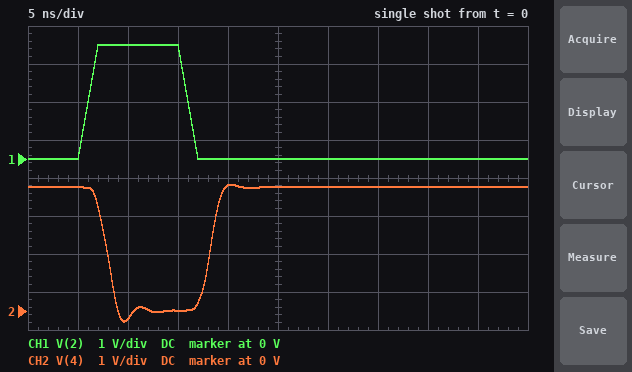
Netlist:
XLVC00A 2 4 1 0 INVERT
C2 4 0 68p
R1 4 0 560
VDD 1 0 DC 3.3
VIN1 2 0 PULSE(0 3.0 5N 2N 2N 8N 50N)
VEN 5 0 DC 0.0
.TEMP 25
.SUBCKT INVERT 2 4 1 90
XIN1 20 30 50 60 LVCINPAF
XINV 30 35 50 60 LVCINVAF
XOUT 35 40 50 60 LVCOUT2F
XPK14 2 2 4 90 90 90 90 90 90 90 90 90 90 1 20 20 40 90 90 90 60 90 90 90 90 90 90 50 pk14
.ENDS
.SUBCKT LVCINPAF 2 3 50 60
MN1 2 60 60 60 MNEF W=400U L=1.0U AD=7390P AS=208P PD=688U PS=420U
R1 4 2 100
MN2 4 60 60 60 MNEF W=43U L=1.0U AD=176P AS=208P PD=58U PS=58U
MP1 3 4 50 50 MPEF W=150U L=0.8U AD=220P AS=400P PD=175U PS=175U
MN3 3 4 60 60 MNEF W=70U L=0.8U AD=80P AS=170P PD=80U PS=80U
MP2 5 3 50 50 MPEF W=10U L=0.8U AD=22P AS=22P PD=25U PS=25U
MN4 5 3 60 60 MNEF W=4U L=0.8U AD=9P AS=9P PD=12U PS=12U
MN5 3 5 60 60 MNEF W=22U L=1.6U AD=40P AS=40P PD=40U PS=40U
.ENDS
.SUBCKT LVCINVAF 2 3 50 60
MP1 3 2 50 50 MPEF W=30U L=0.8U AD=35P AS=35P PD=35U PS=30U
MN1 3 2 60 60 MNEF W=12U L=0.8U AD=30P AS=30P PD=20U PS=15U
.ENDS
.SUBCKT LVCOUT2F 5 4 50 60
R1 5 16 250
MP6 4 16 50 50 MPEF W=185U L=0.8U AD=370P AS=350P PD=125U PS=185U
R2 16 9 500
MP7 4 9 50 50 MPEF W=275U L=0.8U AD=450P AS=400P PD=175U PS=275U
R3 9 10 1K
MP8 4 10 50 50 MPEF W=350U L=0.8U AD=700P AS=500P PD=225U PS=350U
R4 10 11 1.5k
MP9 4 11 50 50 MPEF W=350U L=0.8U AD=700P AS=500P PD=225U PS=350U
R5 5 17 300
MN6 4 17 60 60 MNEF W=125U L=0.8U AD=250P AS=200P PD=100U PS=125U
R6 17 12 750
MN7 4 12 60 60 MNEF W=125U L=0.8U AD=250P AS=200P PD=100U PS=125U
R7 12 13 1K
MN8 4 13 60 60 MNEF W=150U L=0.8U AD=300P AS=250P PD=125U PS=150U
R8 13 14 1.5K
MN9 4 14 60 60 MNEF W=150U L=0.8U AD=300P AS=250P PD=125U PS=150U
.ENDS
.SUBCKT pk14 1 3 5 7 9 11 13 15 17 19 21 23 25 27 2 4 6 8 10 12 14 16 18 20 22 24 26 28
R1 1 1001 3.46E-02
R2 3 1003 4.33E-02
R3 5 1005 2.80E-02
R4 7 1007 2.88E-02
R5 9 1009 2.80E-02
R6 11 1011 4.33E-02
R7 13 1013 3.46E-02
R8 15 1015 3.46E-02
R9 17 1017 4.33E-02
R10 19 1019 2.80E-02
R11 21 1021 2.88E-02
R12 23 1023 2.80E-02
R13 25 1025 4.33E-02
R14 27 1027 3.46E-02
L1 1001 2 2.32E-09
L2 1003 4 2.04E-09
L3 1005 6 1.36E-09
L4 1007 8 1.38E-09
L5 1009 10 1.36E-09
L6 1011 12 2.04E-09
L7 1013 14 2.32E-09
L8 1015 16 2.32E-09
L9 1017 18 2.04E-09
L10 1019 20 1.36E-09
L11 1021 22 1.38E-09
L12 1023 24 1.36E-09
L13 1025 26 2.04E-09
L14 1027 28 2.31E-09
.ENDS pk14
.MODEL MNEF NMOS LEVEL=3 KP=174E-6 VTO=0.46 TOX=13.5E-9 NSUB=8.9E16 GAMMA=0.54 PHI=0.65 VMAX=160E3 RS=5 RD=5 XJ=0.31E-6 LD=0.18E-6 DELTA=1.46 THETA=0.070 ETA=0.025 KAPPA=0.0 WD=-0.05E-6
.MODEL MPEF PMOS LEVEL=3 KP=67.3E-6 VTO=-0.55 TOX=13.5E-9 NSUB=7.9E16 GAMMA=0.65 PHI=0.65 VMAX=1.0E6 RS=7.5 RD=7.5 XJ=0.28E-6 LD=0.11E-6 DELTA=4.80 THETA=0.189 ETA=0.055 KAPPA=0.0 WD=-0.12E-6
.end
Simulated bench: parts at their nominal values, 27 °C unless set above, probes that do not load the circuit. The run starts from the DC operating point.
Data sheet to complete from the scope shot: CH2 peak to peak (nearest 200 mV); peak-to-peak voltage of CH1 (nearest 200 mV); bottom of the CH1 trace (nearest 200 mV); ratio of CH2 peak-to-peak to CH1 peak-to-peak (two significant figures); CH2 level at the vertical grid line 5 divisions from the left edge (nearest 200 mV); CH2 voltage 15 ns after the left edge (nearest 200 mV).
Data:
3.6 V
3.0 V
0 V
1.2
3.2 V
0 V
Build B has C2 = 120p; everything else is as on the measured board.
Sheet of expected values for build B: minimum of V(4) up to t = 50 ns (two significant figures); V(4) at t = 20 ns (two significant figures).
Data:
-230 mV
2.7 V
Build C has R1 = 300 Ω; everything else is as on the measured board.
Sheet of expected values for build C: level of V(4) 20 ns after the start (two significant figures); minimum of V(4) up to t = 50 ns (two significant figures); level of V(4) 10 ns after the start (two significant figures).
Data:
3.3 V
-270 mV
-190 mV
